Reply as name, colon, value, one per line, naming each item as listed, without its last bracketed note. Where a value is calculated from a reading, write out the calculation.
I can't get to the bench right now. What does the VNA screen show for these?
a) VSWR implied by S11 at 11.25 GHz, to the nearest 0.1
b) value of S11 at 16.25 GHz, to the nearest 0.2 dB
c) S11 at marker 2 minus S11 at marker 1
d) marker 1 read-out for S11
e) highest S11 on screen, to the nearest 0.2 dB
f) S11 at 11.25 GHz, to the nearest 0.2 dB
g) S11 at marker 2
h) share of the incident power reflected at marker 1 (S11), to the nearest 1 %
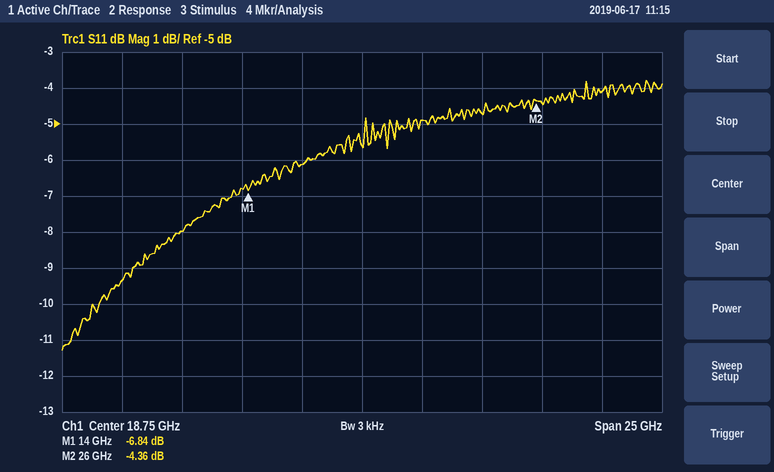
VSWR implied by S11 at 11.25 GHz, to the nearest 0.1: |Γ| = 10^(-8/20) = 0.3981; VSWR = (1 + 0.3981)/(1 − 0.3981) ≈ 2.3
value of S11 at 16.25 GHz, to the nearest 0.2 dB: -6.2 dB
S11 at marker 2 minus S11 at marker 1: -4.36 − (-6.84) = 2.48 dB
marker 1 read-out for S11: -6.84 dB
highest S11 on screen, to the nearest 0.2 dB: -3.8 dB
S11 at 11.25 GHz, to the nearest 0.2 dB: -8.0 dB
S11 at marker 2: -4.36 dB
share of the incident power reflected at marker 1 (S11), to the nearest 1 %: 10^(-6.84/10) ≈ 21 %
